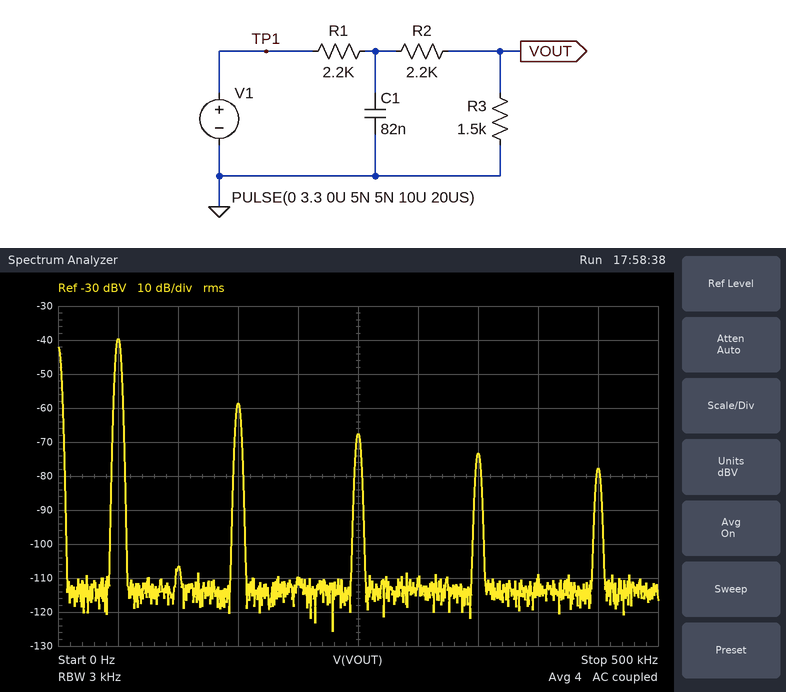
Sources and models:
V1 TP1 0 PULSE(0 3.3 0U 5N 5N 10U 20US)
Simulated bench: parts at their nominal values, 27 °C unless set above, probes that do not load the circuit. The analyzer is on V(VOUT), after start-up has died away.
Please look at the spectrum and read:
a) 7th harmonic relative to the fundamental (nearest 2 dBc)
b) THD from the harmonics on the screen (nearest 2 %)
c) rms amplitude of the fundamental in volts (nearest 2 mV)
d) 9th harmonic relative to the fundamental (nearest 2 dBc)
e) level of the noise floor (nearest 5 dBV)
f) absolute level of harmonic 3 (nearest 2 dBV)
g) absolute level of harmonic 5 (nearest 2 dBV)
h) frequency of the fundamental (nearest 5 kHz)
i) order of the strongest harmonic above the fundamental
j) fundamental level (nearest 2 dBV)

-34 dBc
12 %
10 mV
-38 dBc
-115 dBV
-58 dBV
-68 dBV
50 kHz
3
-40 dBV
